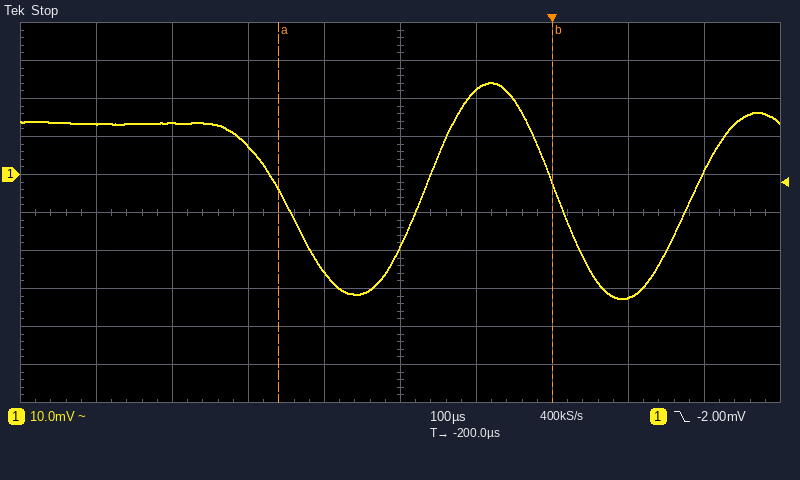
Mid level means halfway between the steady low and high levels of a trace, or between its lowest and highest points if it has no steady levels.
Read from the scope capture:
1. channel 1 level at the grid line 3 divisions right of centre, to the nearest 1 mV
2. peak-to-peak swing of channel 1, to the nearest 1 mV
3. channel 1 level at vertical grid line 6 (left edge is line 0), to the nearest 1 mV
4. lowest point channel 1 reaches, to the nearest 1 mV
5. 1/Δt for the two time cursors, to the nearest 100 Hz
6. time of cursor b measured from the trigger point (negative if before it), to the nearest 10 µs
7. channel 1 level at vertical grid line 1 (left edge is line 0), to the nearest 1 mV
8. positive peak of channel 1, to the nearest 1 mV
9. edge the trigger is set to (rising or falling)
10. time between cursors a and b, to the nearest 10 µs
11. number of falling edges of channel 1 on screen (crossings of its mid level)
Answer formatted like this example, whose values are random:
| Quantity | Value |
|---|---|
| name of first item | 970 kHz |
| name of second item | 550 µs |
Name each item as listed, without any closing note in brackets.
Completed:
| Quantity | Value |
|---|---|
| channel 1 level at the grid line 3 divisions right of centre, to the nearest 1 mV | -32 mV |
| peak-to-peak swing of channel 1, to the nearest 1 mV | 57 mV |
| channel 1 level at vertical grid line 6 (left edge is line 0), to the nearest 1 mV | 22 mV |
| lowest point channel 1 reaches, to the nearest 1 mV | -33 mV |
| 1/Δt for the two time cursors, to the nearest 100 Hz | 2.8 kHz |
| time of cursor b measured from the trigger point (negative if before it), to the nearest 10 µs | 0 µs |
| channel 1 level at vertical grid line 1 (left edge is line 0), to the nearest 1 mV | 13 mV |
| positive peak of channel 1, to the nearest 1 mV | 24 mV |
| edge the trigger is set to | falling |
| time between cursors a and b, to the nearest 10 µs | 360 µs |
| number of falling edges of channel 1 on screen | 2 |
